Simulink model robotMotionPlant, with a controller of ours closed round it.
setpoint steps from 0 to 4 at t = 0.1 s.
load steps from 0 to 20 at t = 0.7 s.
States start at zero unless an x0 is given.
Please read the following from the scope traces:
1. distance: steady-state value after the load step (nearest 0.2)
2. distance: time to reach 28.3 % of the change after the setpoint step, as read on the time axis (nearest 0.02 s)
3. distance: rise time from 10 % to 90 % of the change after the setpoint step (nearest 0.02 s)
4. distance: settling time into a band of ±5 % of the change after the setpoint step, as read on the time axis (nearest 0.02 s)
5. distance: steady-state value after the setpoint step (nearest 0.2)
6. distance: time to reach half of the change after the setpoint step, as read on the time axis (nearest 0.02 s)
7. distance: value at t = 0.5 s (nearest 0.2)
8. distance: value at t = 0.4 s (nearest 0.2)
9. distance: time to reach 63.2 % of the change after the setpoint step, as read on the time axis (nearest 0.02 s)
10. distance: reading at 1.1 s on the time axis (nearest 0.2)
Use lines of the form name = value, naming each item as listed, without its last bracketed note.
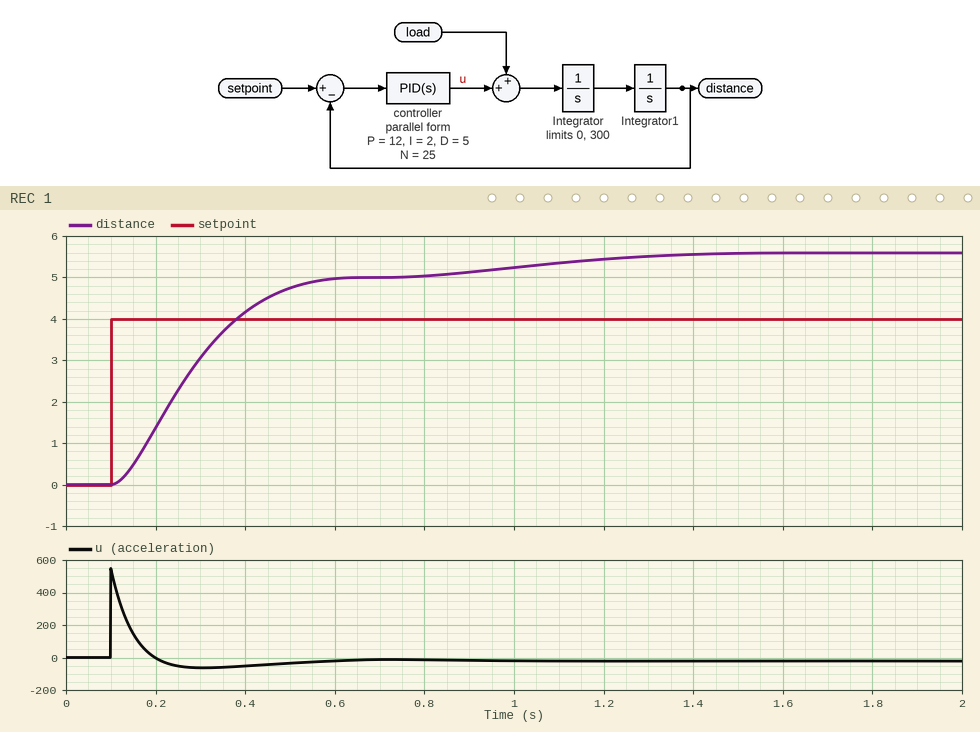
distance: steady-state value after the load step = 5.6
distance: time to reach 28.3 % of the change after the setpoint step, as read on the time axis = 0.20 s
distance: rise time from 10 % to 90 % of the change after the setpoint step = 0.30 s
distance: settling time into a band of ±5 % of the change after the setpoint step, as read on the time axis = 0.50 s
distance: steady-state value after the setpoint step = 5.0
distance: time to reach half of the change after the setpoint step, as read on the time axis = 0.26 s
distance: value at t = 0.5 s = 4.8
distance: value at t = 0.4 s = 4.2
distance: time to reach 63.2 % of the change after the setpoint step, as read on the time axis = 0.30 s
distance: reading at 1.1 s on the time axis = 5.4
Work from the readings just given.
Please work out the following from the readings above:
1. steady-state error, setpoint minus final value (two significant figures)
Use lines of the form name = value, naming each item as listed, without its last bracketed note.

steady-state error, setpoint minus final value = -1.0
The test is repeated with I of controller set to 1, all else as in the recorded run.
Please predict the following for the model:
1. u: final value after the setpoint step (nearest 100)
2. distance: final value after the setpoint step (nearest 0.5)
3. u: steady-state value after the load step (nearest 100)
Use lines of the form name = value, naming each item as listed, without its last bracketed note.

u: final value after the setpoint step = 0
distance: final value after the setpoint step = 5.0
u: steady-state value after the load step = 0
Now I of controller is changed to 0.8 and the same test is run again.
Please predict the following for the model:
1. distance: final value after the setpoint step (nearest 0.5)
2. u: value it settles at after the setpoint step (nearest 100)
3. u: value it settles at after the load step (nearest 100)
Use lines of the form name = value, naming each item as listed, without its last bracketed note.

distance: final value after the setpoint step = 5.0
u: value it settles at after the setpoint step = 0
u: value it settles at after the load step = 0
